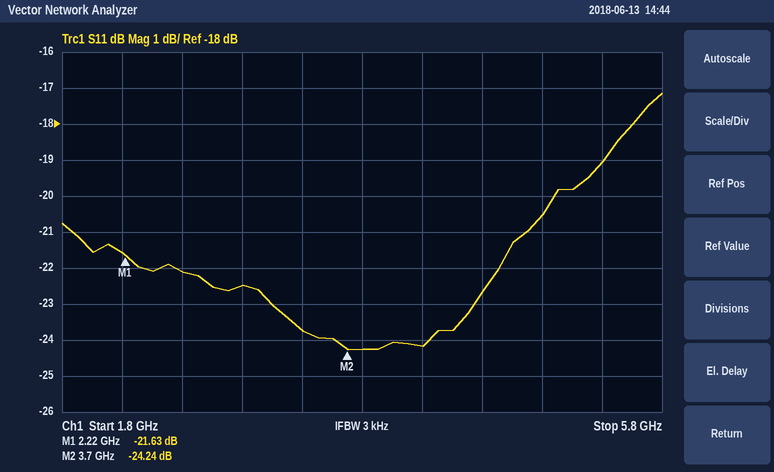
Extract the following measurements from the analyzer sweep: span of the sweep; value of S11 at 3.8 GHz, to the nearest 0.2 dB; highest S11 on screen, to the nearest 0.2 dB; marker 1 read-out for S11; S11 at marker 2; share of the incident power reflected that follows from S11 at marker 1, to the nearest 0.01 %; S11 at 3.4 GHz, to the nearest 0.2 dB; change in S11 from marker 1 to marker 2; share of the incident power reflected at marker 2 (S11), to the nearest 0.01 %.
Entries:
4 GHz
-24.2 dB
-17.2 dB
-21.63 dB
-24.24 dB
0.69 %
-23.8 dB
-2.61 dB
0.38 %
